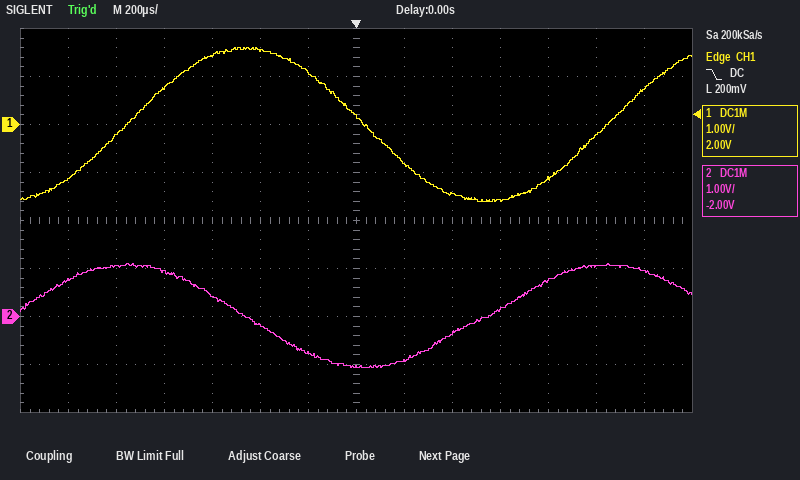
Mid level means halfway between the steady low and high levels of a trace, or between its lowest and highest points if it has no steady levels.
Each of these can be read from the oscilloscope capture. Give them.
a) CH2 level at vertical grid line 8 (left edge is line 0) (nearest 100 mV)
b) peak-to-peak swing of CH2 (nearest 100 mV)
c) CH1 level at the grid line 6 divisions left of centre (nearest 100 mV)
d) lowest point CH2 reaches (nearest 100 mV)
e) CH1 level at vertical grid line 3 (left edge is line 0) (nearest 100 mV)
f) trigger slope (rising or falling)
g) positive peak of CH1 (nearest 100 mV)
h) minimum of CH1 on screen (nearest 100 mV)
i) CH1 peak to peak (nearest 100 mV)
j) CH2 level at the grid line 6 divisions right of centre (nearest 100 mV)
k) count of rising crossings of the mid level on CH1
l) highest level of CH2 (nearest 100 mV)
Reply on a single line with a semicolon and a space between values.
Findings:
-900 mV; 2.2 V; -1.1 V; -1.1 V; 800 mV; falling; 1.6 V; -1.6 V; 3.2 V; 900 mV; 2; 1.1 V
